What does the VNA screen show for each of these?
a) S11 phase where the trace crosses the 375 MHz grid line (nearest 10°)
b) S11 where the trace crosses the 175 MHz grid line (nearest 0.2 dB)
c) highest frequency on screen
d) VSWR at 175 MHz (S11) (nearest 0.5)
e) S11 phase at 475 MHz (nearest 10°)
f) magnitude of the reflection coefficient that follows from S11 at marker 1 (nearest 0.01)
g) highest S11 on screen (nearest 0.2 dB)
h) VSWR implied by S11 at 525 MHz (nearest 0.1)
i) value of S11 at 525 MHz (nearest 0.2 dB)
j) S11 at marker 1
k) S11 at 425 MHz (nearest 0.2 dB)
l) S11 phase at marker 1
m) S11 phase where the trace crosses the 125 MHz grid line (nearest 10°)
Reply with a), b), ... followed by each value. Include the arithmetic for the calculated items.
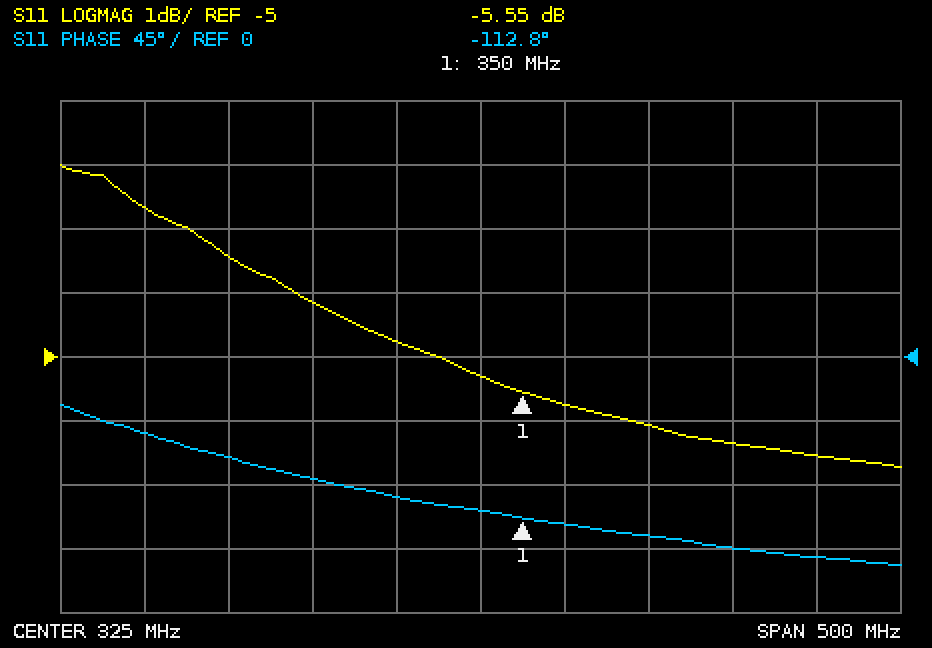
a) -120°
b) -3.4 dB
c) 575 MHz
d) |Γ| = 10^(-3.4/20) = 0.6761; VSWR = (1 + 0.6761)/(1 − 0.6761) ≈ 5.17, so 5.0 to the nearest 0.5
e) -130°
f) 10^(-5.55/20) ≈ 0.53
g) -2.0 dB
h) |Γ| = 10^(-6.6/20) = 0.4677; VSWR = (1 + 0.4677)/(1 − 0.4677) ≈ 2.8
i) -6.6 dB
j) -5.55 dB
k) -6.0 dB
l) -112.8°
m) -50°
